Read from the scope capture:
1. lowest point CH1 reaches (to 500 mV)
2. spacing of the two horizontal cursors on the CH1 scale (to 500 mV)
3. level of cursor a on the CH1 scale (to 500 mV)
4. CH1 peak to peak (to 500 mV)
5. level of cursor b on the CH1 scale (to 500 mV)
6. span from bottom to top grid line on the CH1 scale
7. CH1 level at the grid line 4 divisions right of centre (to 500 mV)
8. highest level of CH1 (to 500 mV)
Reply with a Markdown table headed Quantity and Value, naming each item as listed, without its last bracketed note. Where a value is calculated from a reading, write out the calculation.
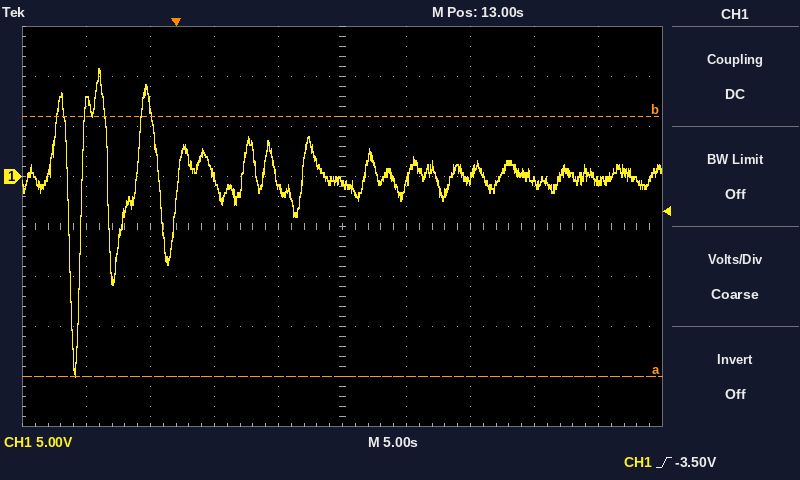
| Quantity | Value |
|---|---|
| lowest point CH1 reaches | -20.0 V |
| spacing of the two horizontal cursors on the CH1 scale | 26.0 V |
| level of cursor a on the CH1 scale | -20.0 V |
| CH1 peak to peak | 11.0 V − (-20.0 V) = 31.0 V |
| level of cursor b on the CH1 scale | 6.0 V |
| span from bottom to top grid line on the CH1 scale | 40 V |
| CH1 level at the grid line 4 divisions right of centre | -500 mV |
| highest level of CH1 | 11.0 V |
